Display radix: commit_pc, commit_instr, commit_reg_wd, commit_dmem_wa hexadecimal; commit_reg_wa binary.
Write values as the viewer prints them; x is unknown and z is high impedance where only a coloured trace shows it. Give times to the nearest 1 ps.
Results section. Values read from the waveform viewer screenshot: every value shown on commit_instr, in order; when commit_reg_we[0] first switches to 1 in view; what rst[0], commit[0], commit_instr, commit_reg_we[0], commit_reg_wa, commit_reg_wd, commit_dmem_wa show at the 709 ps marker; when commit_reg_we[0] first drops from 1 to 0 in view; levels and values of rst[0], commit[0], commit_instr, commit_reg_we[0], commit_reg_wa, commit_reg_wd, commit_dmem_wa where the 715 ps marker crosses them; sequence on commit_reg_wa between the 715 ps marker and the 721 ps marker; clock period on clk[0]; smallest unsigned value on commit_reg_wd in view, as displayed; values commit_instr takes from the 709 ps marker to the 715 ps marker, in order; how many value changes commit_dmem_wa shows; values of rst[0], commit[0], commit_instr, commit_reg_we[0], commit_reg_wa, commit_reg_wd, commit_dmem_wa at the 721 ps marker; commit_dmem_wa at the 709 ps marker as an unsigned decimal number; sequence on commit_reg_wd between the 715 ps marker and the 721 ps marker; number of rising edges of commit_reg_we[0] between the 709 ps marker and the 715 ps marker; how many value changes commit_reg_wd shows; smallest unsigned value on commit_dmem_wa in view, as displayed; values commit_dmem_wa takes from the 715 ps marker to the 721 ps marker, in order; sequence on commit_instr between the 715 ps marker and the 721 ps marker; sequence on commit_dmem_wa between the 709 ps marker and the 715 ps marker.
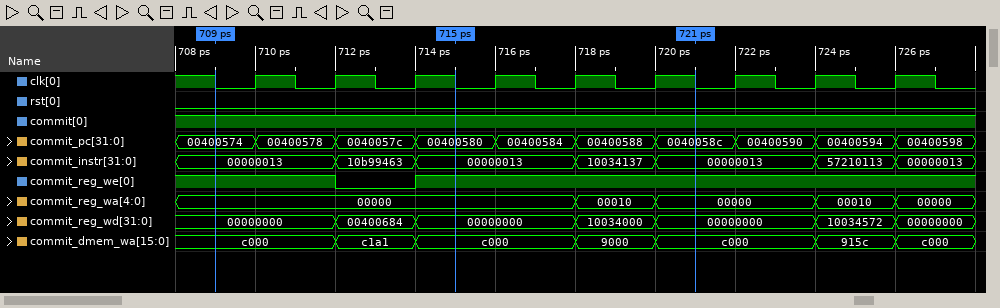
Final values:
00000013, 10b99463, 00000013, 10034137, 00000013, 57210113, 00000013
714 ps
rst[0]=0, commit[0]=1, commit_instr=00000013, commit_reg_we[0]=1, commit_reg_wa=00000, commit_reg_wd=00000000, commit_dmem_wa=c000
712 ps
rst[0]=0, commit[0]=1, commit_instr=00000013, commit_reg_we[0]=1, commit_reg_wa=00000, commit_reg_wd=00000000, commit_dmem_wa=c000
00000, 00010, 00000
2 ps
00000000
00000013, 10b99463, 00000013
6
rst[0]=0, commit[0]=1, commit_instr=00000013, commit_reg_we[0]=1, commit_reg_wa=00000, commit_reg_wd=00000000, commit_dmem_wa=c000
49152
00000000, 10034000, 00000000
1
6
9000
c000, 9000, c000
00000013, 10034137, 00000013
c000, c1a1, c000
